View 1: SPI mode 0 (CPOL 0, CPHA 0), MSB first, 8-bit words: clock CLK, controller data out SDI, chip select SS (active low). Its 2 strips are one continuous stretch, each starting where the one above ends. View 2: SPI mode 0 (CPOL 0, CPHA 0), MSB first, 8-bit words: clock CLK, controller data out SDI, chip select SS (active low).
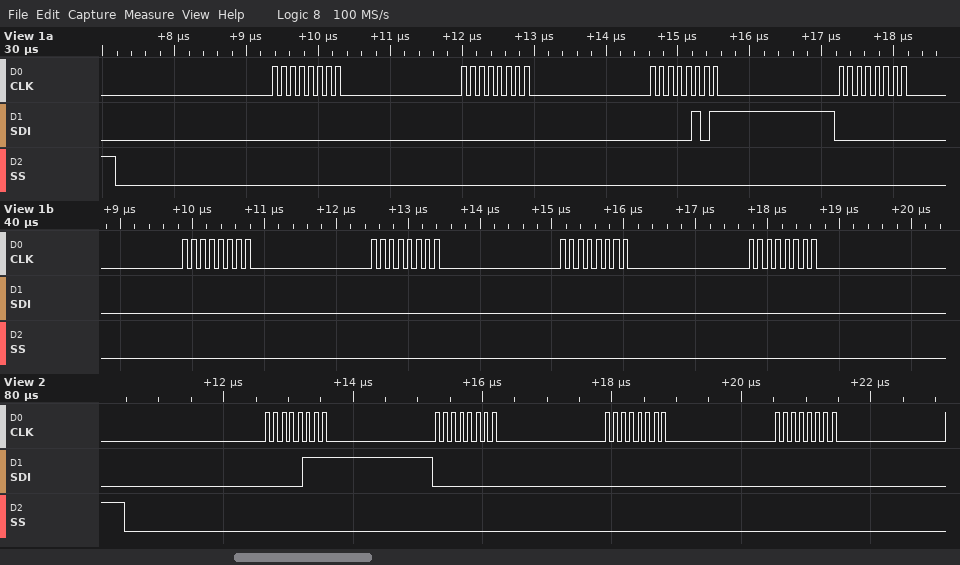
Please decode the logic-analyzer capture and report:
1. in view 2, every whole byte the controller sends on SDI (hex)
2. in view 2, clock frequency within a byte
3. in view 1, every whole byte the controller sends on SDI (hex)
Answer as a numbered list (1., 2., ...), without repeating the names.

1. 07 00 00 00
2. 8 MHz
3. 0x00 0x00 0x05 0x00 0x00 0x00 0x00 0x00
